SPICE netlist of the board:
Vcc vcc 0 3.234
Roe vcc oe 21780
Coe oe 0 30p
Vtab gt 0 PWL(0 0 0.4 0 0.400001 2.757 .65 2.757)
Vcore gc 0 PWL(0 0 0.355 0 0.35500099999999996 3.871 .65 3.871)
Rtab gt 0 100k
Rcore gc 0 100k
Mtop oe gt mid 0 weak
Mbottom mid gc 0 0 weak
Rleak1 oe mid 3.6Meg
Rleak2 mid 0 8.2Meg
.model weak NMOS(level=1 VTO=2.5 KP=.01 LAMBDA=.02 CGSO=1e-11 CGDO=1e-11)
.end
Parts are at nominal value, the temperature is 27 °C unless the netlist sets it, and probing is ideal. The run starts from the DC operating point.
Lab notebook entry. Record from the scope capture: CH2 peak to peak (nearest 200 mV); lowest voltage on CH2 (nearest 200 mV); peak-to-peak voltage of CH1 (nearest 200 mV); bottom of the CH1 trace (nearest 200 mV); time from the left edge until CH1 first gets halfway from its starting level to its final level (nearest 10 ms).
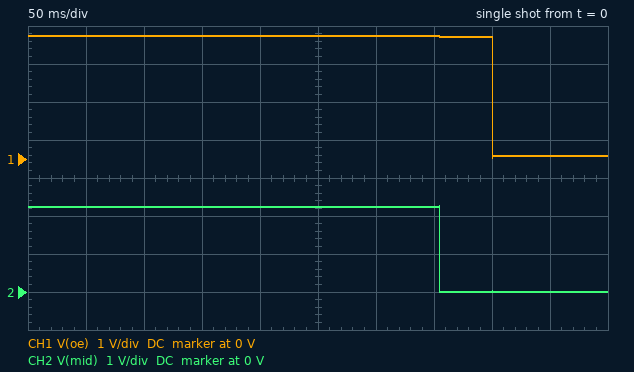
2.2 V
0 V
3.2 V
0 V
400 ms
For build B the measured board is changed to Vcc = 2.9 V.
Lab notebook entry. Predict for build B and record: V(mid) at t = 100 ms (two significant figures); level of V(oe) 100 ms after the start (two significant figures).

2.0 V
2.9 V
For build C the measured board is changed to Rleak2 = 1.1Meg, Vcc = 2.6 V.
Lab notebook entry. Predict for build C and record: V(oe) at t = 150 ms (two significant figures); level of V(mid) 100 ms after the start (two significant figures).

2.6 V
610 mV
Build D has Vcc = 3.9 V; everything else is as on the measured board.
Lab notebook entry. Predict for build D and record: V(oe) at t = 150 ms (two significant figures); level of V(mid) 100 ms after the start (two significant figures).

3.9 V
2.7 V
